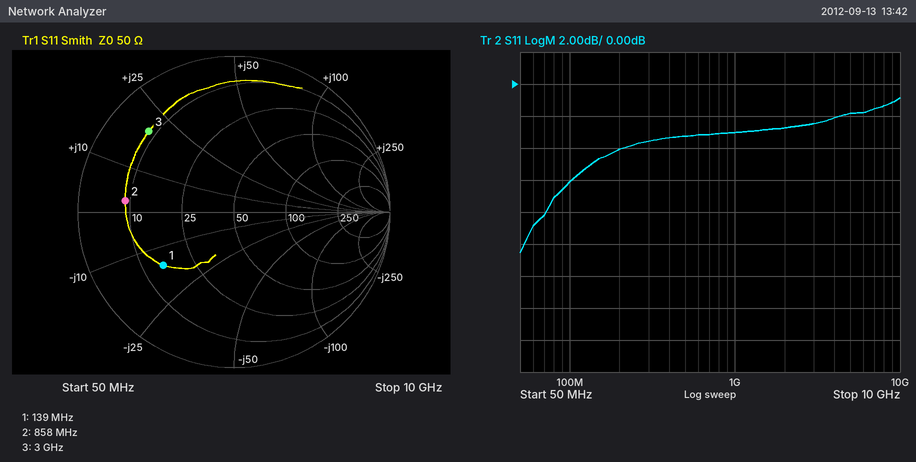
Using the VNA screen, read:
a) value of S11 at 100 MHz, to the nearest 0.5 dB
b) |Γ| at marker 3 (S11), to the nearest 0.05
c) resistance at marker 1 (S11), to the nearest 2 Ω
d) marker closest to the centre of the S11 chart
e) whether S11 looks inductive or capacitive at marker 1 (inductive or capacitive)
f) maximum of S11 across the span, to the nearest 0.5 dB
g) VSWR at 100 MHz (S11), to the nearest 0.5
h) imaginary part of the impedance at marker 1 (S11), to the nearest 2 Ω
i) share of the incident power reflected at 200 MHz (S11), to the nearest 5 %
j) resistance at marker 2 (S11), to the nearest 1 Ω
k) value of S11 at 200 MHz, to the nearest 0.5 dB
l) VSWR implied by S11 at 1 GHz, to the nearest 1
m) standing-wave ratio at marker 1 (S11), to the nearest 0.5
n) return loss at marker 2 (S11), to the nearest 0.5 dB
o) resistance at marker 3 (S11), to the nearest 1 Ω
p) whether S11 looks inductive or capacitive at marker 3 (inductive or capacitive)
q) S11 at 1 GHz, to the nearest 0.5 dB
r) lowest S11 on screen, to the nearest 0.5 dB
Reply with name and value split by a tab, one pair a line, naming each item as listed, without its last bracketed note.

value of S11 at 100 MHz, to the nearest 0.5 dB	-6.0 dB
|Γ| at marker 3 (S11), to the nearest 0.05	0.75
resistance at marker 1 (S11), to the nearest 2 Ω	16 Ω
marker closest to the centre of the S11 chart	marker 1
whether S11 looks inductive or capacitive at marker 1	capacitive
maximum of S11 across the span, to the nearest 0.5 dB	-1.0 dB
VSWR at 100 MHz (S11), to the nearest 0.5	3.0
imaginary part of the impedance at marker 1 (S11), to the nearest 2 Ω	-16 Ω
share of the incident power reflected at 200 MHz (S11), to the nearest 5 %	40 %
resistance at marker 2 (S11), to the nearest 1 Ω	9 Ω
value of S11 at 200 MHz, to the nearest 0.5 dB	-4.0 dB
VSWR implied by S11 at 1 GHz, to the nearest 1	6
standing-wave ratio at marker 1 (S11), to the nearest 0.5	3.5
return loss at marker 2 (S11), to the nearest 0.5 dB	3.0 dB
resistance at marker 3 (S11), to the nearest 1 Ω	8 Ω
whether S11 looks inductive or capacitive at marker 3	inductive
S11 at 1 GHz, to the nearest 0.5 dB	-3.0 dB
lowest S11 on screen, to the nearest 0.5 dB	-10.5 dB
